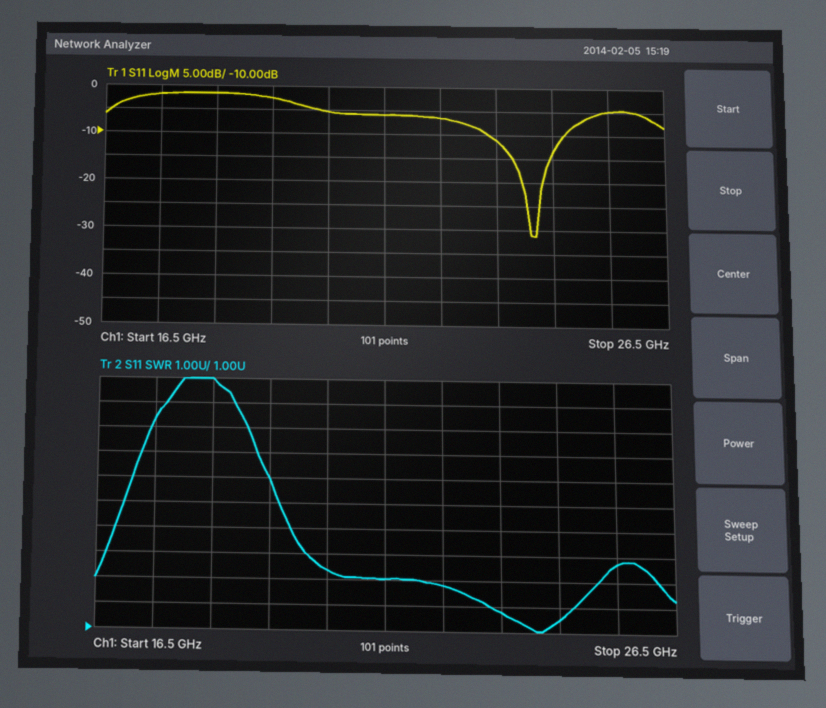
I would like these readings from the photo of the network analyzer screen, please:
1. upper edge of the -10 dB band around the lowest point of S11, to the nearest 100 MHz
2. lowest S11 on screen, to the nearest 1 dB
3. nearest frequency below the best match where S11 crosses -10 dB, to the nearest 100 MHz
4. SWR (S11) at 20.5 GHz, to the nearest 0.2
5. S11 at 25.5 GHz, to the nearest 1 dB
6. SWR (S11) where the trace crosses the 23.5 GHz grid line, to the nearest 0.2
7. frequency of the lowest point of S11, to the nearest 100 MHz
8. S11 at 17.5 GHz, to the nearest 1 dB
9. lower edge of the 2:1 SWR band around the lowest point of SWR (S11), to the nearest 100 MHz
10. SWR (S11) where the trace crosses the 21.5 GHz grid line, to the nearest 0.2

24.7 GHz
-31 dB
23.4 GHz
3.4
-5 dB
1.8
24.2 GHz
-2 dB
23.3 GHz
3.0
